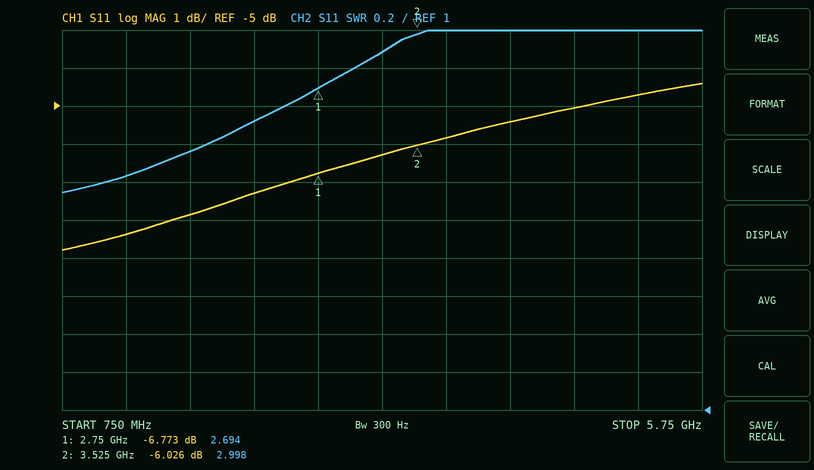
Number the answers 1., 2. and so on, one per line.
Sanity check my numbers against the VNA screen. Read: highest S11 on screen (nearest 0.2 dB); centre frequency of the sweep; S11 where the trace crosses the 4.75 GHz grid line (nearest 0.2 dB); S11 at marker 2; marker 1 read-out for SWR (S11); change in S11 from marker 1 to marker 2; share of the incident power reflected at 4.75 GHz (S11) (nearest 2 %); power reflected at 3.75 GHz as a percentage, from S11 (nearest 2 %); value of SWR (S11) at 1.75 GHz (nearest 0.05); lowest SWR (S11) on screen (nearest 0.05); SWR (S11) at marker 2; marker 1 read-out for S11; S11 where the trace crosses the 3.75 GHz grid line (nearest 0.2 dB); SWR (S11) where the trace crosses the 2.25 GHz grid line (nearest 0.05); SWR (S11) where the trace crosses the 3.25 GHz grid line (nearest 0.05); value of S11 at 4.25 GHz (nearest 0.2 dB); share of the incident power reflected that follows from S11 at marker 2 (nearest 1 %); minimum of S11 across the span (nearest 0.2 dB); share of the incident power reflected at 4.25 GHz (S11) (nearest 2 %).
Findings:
1. -4.4 dB
2. 3.25 GHz
3. -5.0 dB
4. -6.026 dB
5. 2.694
6. 0.747 dB
7. 32 %
8. 26 %
9. 2.35
10. 2.15
11. 2.998
12. -6.773 dB
13. -5.8 dB
14. 2.50
15. 2.90
16. -5.4 dB
17. 25 %
18. -8.8 dB
19. 28 %
